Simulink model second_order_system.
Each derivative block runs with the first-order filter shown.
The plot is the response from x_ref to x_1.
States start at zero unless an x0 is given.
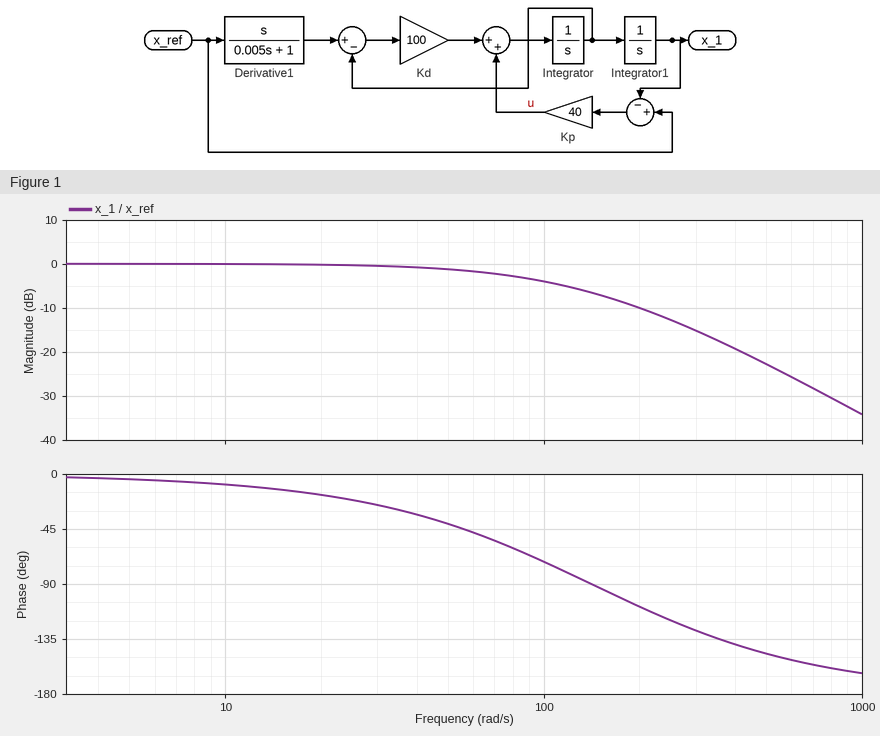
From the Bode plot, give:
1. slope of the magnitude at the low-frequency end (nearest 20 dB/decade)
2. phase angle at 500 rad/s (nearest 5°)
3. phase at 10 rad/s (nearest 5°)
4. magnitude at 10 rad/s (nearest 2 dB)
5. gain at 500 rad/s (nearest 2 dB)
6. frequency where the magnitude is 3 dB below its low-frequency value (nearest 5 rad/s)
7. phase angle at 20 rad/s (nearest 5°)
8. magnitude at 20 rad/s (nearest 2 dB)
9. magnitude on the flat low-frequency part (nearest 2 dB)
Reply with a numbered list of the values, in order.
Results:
1. 0 dB/decade
2. -145°
3. -10°
4. 0 dB
5. -22 dB
6. 85 rad/s
7. -15°
8. 0 dB
9. 0 dB
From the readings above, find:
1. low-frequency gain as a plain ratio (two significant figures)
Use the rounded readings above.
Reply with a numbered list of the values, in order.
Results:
1. 1.0
